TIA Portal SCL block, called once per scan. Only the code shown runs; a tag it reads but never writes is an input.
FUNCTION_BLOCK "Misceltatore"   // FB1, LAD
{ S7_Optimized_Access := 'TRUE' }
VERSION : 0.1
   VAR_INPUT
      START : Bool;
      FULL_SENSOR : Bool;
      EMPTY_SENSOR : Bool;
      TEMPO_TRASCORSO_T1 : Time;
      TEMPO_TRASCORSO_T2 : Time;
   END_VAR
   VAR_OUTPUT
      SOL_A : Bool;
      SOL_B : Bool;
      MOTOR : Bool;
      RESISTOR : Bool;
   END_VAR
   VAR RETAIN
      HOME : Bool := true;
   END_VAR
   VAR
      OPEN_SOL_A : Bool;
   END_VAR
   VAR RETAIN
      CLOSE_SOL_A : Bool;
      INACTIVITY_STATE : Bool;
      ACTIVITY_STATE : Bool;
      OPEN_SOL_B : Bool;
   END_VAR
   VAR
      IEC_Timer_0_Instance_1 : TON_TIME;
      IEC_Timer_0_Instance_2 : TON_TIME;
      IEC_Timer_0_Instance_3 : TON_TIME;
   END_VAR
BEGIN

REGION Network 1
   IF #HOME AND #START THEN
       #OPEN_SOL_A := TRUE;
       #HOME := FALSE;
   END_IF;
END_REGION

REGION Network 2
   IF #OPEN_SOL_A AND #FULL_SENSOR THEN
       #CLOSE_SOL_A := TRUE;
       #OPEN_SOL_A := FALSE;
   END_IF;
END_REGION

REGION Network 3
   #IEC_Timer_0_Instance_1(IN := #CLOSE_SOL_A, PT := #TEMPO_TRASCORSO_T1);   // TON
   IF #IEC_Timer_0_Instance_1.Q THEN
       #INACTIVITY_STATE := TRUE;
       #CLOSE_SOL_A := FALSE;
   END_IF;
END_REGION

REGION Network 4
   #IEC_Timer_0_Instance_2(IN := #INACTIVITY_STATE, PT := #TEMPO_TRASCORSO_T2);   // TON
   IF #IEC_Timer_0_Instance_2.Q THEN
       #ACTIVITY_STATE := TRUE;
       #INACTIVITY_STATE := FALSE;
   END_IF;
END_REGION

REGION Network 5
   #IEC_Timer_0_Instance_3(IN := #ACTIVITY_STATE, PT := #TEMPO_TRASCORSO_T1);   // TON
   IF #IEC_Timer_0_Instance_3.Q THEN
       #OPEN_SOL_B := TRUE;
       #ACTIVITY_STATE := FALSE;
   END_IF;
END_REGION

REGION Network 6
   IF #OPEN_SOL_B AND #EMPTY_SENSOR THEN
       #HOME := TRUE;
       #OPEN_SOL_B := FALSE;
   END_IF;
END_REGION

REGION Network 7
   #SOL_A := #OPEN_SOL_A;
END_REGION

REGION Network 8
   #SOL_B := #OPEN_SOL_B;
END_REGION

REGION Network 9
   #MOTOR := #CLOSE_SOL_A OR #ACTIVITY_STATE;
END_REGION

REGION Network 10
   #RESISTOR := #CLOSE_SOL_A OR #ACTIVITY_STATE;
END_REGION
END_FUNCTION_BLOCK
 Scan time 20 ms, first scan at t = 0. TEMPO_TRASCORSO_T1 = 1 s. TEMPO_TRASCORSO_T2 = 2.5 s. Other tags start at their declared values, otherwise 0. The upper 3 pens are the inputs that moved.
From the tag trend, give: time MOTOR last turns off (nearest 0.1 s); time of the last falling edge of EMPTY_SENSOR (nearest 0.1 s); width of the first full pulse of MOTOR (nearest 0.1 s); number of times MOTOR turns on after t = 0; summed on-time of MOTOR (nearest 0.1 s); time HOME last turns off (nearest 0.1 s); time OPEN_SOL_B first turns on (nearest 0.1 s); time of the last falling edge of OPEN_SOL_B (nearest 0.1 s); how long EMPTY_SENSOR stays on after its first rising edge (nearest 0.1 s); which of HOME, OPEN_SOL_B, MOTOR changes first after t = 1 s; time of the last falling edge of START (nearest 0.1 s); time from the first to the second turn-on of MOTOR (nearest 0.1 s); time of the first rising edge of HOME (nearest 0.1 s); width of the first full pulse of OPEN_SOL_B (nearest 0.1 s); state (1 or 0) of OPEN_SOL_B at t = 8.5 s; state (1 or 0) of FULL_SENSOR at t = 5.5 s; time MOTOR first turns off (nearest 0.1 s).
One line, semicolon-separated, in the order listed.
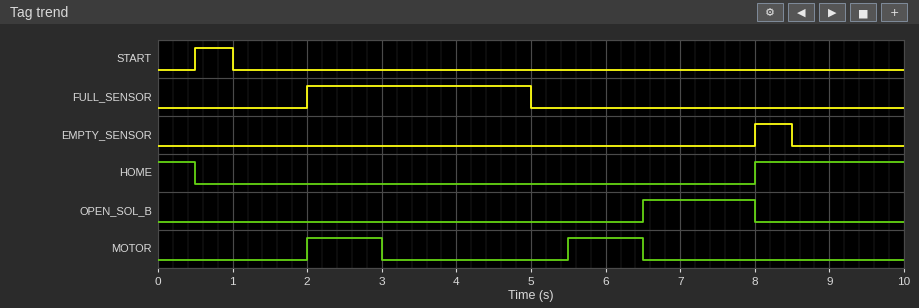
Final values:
6.5 s; 8.5 s; 1.0 s; 2; 2.0 s; 0.5 s; 6.5 s; 8.0 s; 0.5 s; MOTOR; 1.0 s; 3.5 s; 8.0 s; 1.5 s; 0; 0; 3.0 s
